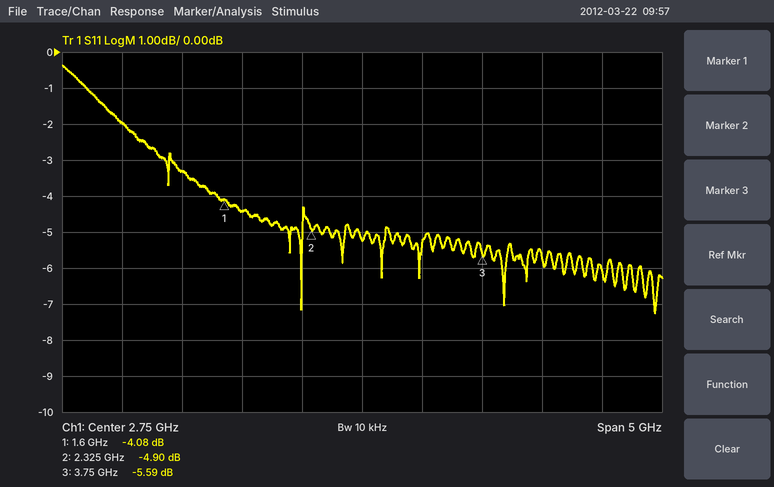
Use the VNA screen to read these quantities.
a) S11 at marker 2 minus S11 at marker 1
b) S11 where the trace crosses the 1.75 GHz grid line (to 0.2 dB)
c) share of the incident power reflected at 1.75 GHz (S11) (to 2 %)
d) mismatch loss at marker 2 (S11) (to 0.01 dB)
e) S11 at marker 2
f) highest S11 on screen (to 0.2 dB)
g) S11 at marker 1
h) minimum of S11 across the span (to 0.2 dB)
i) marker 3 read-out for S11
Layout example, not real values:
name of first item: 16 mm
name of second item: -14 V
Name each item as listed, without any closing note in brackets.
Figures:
S11 at marker 2 minus S11 at marker 1: -0.82 dB
S11 where the trace crosses the 1.75 GHz grid line: -4.4 dB
share of the incident power reflected at 1.75 GHz (S11): 36 %
mismatch loss at marker 2 (S11): 1.70 dB
S11 at marker 2: -4.90 dB
highest S11 on screen: -0.4 dB
S11 at marker 1: -4.08 dB
minimum of S11 across the span: -7.2 dB
marker 3 read-out for S11: -5.59 dB
